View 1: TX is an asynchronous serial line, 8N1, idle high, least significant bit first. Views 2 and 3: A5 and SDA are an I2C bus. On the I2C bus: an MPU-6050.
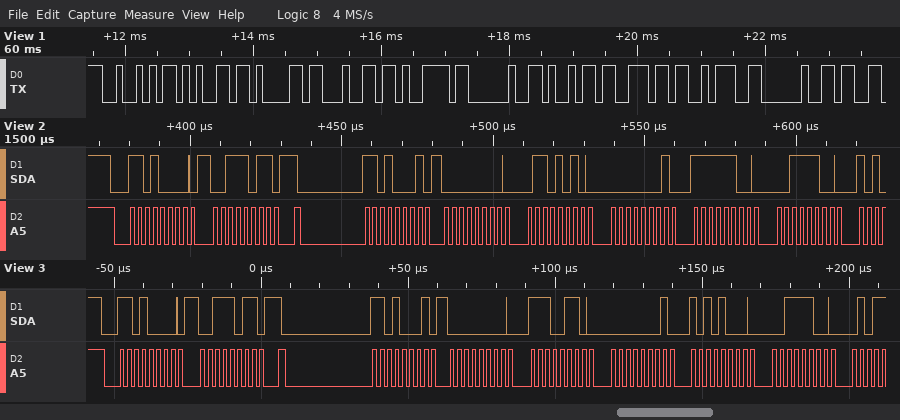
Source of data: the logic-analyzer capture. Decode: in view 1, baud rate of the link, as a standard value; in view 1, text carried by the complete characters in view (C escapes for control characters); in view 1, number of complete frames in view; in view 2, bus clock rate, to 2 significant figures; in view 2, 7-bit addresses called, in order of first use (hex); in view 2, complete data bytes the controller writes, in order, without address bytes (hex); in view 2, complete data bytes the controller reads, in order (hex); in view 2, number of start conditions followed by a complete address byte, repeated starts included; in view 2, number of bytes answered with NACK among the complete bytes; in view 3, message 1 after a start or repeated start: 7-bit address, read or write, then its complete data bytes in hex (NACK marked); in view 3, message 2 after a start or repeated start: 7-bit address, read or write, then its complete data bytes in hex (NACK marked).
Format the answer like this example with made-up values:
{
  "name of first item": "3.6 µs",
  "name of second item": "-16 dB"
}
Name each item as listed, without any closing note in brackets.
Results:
{
  "in view 1, baud rate of the link, as a standard value": "9600 baud",
  "in view 1, text carried by the complete characters in view": "\"Ready in: \"",
  "in view 1, number of complete frames in view": "10",
  "in view 2, bus clock rate, to 2 significant figures": "400 kHz",
  "in view 2, 7-bit addresses called, in order of first use": "0x68",
  "in view 2, complete data bytes the controller writes, in order, without address bytes": "3B",
  "in view 2, complete data bytes the controller reads, in order": "00 6A 01 FC 3C",
  "in view 2, number of start conditions followed by a complete address byte, repeated starts included": "2",
  "in view 2, number of bytes answered with NACK among the complete bytes": "0",
  "in view 3, message 1 after a start or repeated start: 7-bit address, read or write, then its complete data bytes in hex": "0x68 write: 3B",
  "in view 3, message 2 after a start or repeated start: 7-bit address, read or write, then its complete data bytes in hex": "0x68 read: 00 E6 01 A8 3C"
}
